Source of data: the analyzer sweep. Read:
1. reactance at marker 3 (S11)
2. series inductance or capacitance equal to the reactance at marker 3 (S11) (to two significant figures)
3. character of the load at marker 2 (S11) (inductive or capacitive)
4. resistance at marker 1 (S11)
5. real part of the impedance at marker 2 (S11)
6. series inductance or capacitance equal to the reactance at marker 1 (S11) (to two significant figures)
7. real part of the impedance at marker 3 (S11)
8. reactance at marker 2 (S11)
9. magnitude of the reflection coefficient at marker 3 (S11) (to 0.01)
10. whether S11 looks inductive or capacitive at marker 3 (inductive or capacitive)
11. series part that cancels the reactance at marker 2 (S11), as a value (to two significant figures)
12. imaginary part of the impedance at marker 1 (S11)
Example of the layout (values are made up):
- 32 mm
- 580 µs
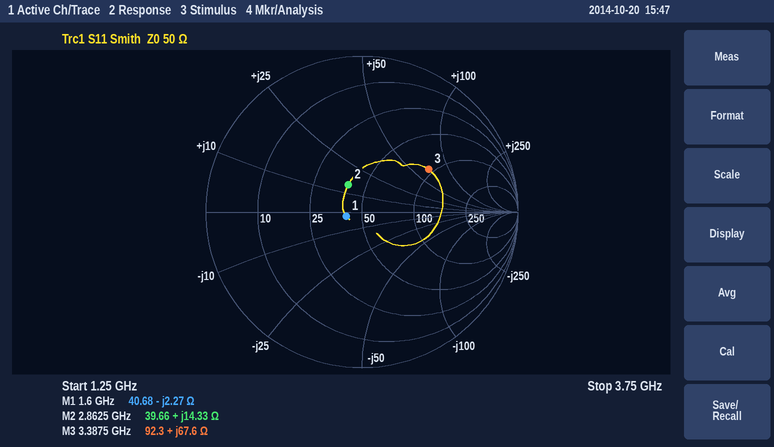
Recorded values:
- +67.6 Ω
- 3.2 nH
- inductive
- 40.68 Ω
- 39.66 Ω
- 44 pF
- 92.3 Ω
- +14.33 Ω
- 0.51
- inductive
- 3.9 pF
- -2.27 Ω
